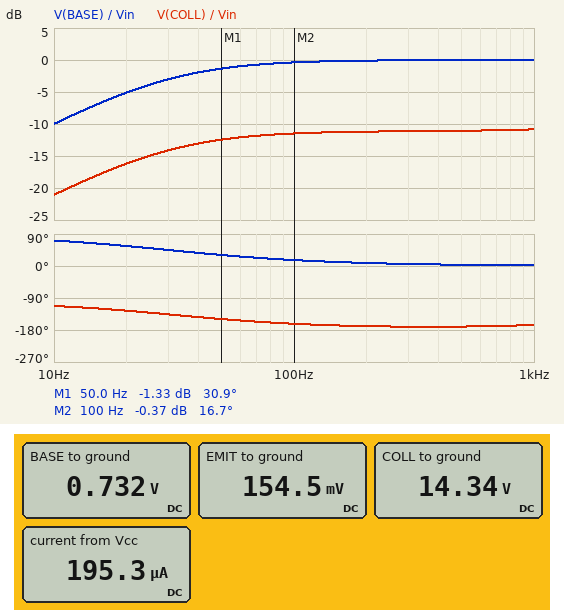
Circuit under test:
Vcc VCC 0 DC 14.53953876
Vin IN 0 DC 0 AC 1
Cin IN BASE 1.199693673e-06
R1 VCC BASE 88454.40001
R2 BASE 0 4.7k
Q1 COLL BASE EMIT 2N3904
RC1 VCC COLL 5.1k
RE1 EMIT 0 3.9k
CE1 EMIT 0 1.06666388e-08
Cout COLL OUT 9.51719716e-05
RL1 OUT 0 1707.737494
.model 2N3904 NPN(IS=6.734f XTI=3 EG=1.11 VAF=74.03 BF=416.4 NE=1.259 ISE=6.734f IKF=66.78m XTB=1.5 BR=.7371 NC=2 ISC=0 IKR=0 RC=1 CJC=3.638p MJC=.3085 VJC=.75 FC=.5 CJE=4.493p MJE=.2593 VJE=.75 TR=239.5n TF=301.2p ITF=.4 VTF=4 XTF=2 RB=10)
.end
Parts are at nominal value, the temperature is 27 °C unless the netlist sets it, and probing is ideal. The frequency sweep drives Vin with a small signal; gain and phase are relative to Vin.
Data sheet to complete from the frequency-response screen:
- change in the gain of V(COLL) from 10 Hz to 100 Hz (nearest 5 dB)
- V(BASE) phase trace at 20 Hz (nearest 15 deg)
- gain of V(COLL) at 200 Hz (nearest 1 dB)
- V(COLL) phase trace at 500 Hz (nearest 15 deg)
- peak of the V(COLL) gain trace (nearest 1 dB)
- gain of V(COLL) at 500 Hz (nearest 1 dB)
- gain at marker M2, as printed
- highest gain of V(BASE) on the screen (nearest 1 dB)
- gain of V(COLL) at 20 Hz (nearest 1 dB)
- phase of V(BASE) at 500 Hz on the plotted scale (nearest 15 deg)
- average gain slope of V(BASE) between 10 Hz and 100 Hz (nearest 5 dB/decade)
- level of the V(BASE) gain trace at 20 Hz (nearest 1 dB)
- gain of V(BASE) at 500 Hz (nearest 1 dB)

10 dB
60 deg
-11 dB
-165 deg
-11 dB
-11 dB
-0.37 dB
0 dB
-16 dB
0 deg
10 dB/decade
-5 dB
0 dB
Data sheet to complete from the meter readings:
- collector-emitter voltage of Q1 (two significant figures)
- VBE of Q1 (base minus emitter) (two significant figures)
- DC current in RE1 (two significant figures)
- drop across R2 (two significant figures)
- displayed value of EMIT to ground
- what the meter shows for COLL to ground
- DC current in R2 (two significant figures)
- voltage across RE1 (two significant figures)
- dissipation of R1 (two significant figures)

14 V
580 mV
40 µA
730 mV
154.5 mV
14.34 V
160 µA
150 mV
2.2 mW
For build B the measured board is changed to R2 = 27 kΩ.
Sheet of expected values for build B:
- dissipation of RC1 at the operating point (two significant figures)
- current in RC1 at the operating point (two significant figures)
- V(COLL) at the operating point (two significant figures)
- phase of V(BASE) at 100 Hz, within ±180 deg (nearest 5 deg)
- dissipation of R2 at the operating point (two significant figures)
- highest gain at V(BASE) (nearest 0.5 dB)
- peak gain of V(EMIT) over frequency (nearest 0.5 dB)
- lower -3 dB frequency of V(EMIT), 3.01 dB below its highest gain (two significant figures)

2.3 mW
670 µA
11 V
5 deg
400 µW
0 dB
0 dB
6.6 Hz
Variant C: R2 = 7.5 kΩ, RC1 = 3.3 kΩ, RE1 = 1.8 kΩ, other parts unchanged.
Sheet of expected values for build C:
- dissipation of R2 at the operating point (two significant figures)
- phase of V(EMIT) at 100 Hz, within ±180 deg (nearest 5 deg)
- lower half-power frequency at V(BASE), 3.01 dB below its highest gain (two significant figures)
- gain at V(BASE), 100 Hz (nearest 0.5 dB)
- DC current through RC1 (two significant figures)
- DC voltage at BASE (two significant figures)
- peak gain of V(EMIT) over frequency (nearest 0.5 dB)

170 µW
10 deg
20 Hz
0 dB
270 µA
1.1 V
-0.5 dB
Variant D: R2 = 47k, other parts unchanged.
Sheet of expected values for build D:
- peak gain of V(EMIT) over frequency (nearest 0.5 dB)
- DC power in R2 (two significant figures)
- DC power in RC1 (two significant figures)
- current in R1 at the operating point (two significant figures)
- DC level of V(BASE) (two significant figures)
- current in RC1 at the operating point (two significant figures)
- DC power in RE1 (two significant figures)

0 dB
490 µW
5.7 mW
110 µA
4.8 V
1.1 mA
4.4 mW
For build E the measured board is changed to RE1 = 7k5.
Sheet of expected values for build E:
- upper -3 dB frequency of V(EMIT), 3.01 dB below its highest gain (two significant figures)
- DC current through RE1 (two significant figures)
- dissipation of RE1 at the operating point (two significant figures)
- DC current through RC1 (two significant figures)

15 kHz
23 µA
3.8 µW
22 µA
